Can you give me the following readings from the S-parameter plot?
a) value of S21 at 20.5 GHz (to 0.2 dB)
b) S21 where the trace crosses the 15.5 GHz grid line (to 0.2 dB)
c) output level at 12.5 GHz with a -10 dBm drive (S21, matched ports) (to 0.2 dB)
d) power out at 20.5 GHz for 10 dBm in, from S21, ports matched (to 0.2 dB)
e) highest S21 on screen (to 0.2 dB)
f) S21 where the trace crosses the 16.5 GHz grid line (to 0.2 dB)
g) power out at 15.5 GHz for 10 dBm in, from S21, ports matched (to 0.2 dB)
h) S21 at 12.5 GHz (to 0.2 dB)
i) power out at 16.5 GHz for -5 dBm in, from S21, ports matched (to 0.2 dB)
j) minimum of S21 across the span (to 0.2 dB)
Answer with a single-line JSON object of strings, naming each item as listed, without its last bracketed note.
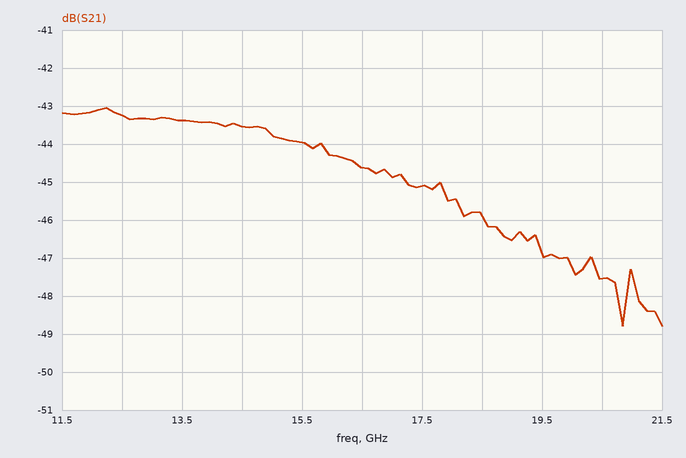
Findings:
{"value of S21 at 20.5 GHz": "-47.6 dB", "S21 where the trace crosses the 15.5 GHz grid line": "-44.0 dB", "output level at 12.5 GHz with a -10 dBm drive (S21, matched ports)": "-53.2 dBm", "power out at 20.5 GHz for 10 dBm in, from S21, ports matched": "-37.6 dBm", "highest S21 on screen": "-43.0 dB", "S21 where the trace crosses the 16.5 GHz grid line": "-44.6 dB", "power out at 15.5 GHz for 10 dBm in, from S21, ports matched": "-34.0 dBm", "S21 at 12.5 GHz": "-43.2 dB", "power out at 16.5 GHz for -5 dBm in, from S21, ports matched": "-49.6 dBm", "minimum of S21 across the span": "-48.8 dB"}
